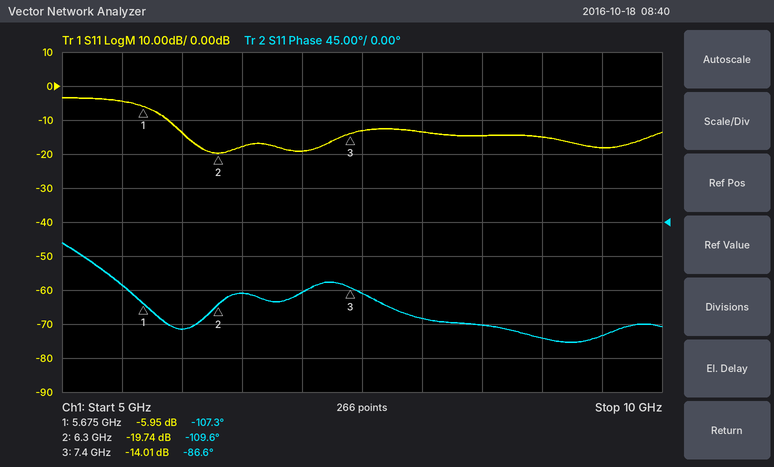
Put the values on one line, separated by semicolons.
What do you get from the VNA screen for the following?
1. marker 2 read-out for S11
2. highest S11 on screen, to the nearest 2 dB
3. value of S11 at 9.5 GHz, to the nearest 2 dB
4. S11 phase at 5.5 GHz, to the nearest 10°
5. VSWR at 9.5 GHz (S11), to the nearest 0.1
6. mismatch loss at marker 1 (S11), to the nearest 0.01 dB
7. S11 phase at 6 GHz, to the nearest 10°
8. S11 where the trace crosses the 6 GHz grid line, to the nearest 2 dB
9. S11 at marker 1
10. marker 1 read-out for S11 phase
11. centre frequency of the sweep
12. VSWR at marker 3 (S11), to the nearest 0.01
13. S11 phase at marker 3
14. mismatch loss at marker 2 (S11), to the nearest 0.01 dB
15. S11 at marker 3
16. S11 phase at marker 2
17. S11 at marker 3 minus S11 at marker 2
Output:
-19.74 dB; -4 dB; -18 dB; -80°; 1.3; 1.27 dB; -140°; -14 dB; -5.95 dB; -107.3°; 7.5 GHz; 1.50; -86.6°; 0.05 dB; -14.01 dB; -109.6°; 5.73 dB
